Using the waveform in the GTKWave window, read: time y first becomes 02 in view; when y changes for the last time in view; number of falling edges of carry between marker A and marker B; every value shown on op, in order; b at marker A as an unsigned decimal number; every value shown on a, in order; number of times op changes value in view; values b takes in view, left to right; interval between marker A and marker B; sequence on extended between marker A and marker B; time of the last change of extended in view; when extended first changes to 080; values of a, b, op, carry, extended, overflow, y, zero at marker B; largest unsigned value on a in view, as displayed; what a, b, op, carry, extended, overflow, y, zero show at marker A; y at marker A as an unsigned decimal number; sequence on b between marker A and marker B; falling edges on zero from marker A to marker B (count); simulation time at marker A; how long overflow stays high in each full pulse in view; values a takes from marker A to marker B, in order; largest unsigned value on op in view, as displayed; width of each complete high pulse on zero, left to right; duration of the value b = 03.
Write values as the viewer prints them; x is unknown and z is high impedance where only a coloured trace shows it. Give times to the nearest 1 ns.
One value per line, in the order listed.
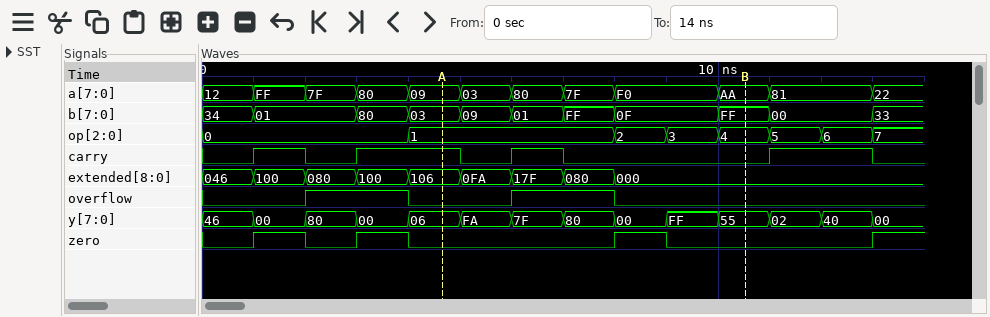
11 ns
13 ns
2
0, 1, 2, 3, 4, 5, 6, 7
3
12, FF, 7F, 80, 09, 03, 80, 7F, F0, AA, 81, 22
7
34, 01, 80, 03, 09, 01, FF, 0F, FF, 00, 33
6 ns
106, 0FA, 17F, 080, 000
8 ns
2 ns
a=AA, b=FF, op=4, carry=0, extended=000, overflow=0, y=55, zero=0
FF
a=09, b=03, op=1, carry=1, extended=106, overflow=0, y=06, zero=0
6
03, 09, 01, FF, 0F, FF
1
5 ns
2 ns, 2 ns
09, 03, 80, 7F, F0, AA
7
1 ns, 1 ns, 1 ns
1 ns
